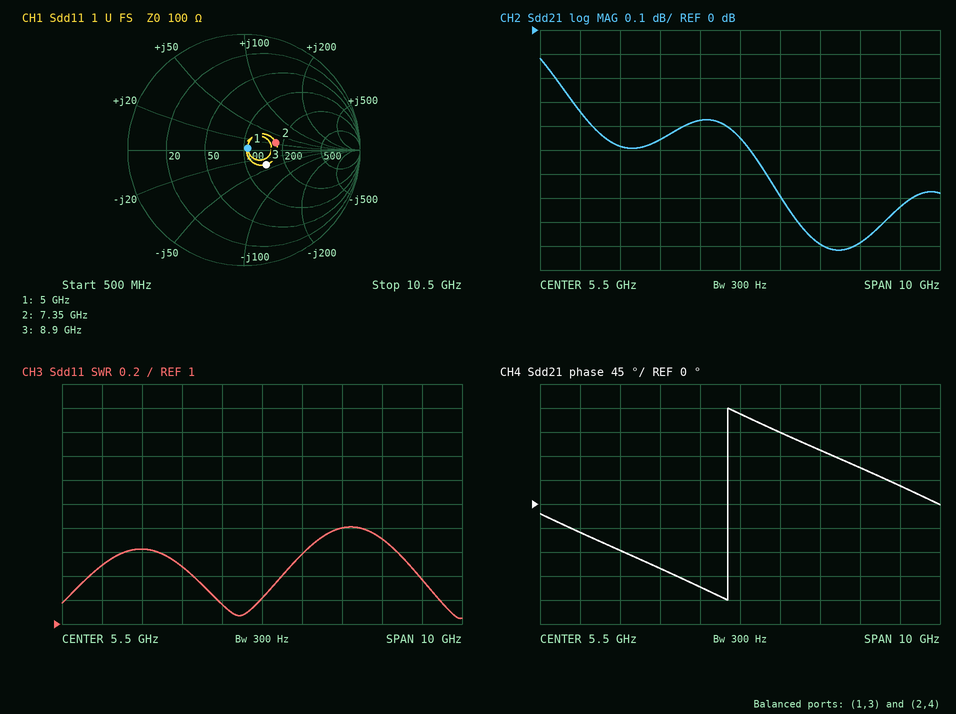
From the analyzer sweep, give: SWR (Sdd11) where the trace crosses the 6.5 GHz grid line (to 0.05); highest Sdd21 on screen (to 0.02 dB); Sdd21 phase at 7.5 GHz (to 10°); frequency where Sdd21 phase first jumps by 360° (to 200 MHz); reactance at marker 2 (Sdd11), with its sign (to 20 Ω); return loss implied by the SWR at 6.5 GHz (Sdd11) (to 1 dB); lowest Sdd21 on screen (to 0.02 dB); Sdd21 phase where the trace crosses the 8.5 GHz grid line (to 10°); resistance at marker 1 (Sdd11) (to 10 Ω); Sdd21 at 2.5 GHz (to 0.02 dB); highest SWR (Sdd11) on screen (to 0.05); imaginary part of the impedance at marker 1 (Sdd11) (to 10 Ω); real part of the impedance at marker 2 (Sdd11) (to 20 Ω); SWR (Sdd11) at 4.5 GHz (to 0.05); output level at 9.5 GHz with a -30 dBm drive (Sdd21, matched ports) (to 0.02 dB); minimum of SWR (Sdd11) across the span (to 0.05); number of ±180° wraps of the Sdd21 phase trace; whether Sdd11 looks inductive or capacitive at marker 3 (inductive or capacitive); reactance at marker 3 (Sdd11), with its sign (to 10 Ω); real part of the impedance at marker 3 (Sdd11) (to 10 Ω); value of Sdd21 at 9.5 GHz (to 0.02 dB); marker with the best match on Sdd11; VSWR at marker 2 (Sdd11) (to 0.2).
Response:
1.60
-0.12 dB
100°
5.2 GHz
+20 Ω
13 dB
-0.92 dB
70°
110 Ω
-0.48 dB
1.80
0 Ω
180 Ω
1.15
-30.74 dBm
1.05
1
capacitive
-40 Ω
140 Ω
-0.74 dB
marker 1
1.8
